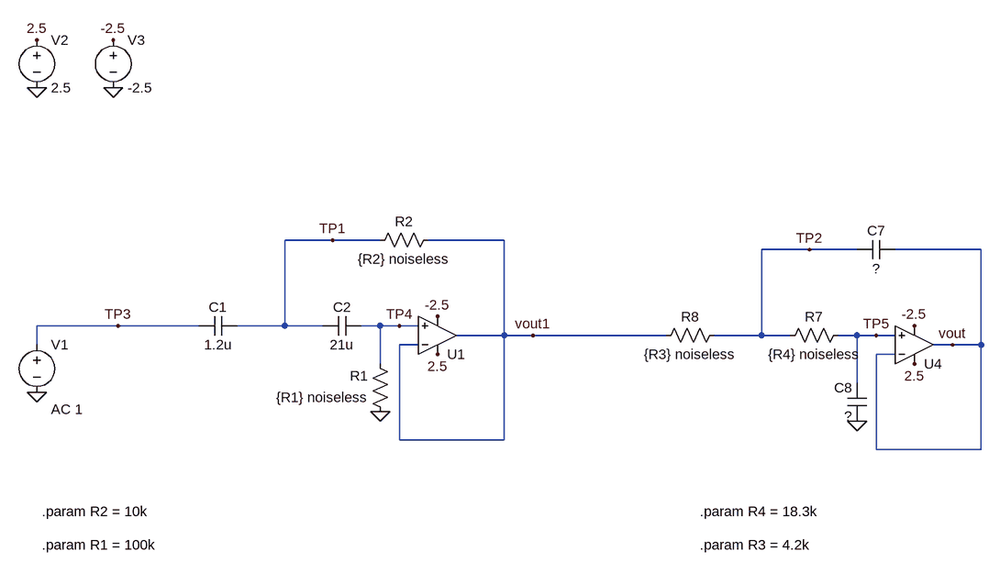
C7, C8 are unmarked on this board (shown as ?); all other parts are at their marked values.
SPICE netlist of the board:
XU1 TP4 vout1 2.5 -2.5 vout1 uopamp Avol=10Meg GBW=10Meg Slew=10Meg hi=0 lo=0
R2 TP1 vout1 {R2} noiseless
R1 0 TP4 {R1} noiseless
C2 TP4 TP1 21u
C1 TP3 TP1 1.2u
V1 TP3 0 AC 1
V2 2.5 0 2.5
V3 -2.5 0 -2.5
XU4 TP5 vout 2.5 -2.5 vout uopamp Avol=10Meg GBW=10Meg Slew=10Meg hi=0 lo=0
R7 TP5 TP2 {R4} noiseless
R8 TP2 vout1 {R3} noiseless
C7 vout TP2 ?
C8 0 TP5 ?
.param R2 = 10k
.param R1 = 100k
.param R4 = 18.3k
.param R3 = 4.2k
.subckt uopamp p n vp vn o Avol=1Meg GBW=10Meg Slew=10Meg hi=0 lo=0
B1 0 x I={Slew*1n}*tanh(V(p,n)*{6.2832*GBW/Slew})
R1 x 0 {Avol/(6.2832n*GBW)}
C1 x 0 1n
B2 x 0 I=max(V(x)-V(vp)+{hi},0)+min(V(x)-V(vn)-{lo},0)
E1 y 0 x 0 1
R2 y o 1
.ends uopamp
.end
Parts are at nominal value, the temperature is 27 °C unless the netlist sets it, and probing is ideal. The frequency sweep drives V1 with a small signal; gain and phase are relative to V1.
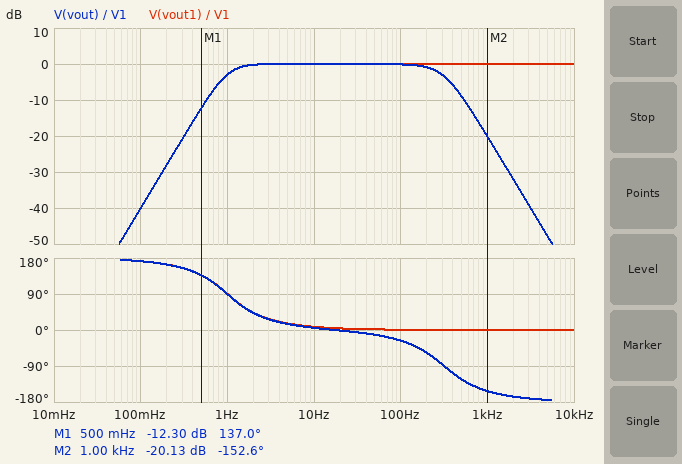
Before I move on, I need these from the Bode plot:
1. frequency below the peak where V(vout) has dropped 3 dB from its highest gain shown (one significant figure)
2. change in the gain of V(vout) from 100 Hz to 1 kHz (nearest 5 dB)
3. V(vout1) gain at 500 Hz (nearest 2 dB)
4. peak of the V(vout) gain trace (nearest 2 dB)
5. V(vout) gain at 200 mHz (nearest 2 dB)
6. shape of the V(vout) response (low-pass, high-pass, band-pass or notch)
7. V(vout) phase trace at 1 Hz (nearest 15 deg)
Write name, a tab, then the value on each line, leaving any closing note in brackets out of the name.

frequency below the peak where V(vout) has dropped 3 dB from its highest gain shown	1 Hz
change in the gain of V(vout) from 100 Hz to 1 kHz	-20 dB
V(vout1) gain at 500 Hz	0 dB
peak of the V(vout) gain trace	0 dB
V(vout) gain at 200 mHz	-28 dB
shape of the V(vout) response	band-pass
V(vout) phase trace at 1 Hz	90 deg
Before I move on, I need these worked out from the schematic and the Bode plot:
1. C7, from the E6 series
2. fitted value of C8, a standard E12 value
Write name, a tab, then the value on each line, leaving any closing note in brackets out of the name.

C7, from the E6 series	100 nF
fitted value of C8, a standard E12 value	33 nF
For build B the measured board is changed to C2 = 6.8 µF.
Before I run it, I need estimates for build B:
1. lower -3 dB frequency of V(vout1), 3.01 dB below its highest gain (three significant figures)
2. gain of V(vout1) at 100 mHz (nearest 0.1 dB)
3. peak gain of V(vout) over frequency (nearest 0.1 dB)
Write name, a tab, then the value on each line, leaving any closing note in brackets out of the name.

lower -3 dB frequency of V(vout1), 3.01 dB below its highest gain	1.49 Hz
gain of V(vout1) at 100 mHz	-49.8 dB
peak gain of V(vout) over frequency	2.0 dB
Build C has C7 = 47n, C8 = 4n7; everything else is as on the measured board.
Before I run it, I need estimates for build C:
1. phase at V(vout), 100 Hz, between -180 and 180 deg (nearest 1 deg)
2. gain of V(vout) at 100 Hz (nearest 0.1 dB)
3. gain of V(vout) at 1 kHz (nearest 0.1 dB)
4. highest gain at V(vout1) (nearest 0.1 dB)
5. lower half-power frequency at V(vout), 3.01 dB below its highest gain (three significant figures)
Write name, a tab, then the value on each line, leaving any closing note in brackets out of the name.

phase at V(vout), 100 Hz, between -180 and 180 deg	-3 deg
gain of V(vout) at 100 Hz	0 dB
gain of V(vout) at 1 kHz	2.6 dB
highest gain at V(vout1)	0 dB
lower half-power frequency at V(vout), 3.01 dB below its highest gain	1.72 Hz
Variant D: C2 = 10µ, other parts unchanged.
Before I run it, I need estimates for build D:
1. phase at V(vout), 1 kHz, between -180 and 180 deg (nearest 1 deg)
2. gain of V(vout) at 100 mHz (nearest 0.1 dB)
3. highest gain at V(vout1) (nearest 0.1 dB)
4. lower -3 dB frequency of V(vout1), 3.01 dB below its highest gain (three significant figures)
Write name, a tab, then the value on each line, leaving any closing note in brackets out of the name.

phase at V(vout), 1 kHz, between -180 and 180 deg	-153 deg
gain of V(vout) at 100 mHz	-46.5 dB
highest gain at V(vout1)	1.1 dB
lower -3 dB frequency of V(vout1), 3.01 dB below its highest gain	1.25 Hz
